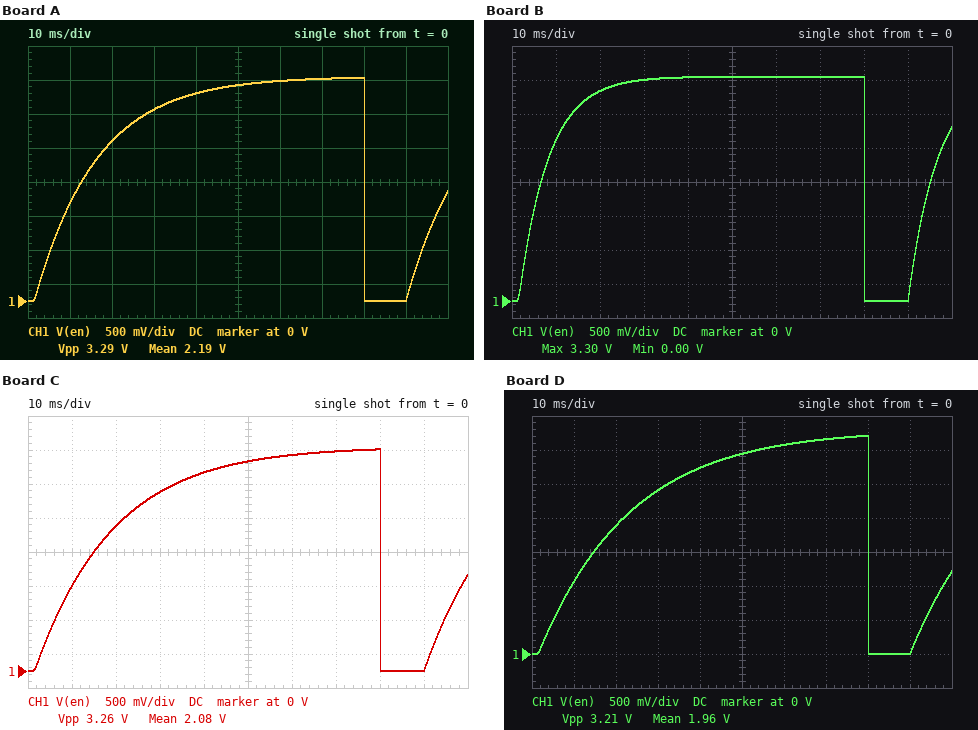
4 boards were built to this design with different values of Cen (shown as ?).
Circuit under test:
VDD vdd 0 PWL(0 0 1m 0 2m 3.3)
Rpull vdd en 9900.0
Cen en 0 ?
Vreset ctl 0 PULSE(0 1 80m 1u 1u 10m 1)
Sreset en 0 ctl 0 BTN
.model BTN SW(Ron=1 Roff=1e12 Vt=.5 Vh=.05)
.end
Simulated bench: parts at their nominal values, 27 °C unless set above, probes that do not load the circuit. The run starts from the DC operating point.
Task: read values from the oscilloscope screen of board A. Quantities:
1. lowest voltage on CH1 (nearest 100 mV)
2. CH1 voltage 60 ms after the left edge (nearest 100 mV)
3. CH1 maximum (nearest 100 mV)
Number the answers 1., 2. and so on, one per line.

1. 0 V
2. 3.2 V
3. 3.3 V
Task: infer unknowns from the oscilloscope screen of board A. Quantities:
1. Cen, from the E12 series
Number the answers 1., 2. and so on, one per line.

1. 1.5 µF
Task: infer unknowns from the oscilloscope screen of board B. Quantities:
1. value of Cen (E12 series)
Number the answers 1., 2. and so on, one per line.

1. 680 nF
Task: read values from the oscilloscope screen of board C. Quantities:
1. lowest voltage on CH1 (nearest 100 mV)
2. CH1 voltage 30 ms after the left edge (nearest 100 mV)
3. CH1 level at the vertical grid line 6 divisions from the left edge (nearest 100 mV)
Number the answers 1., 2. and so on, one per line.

1. 0 V
2. 2.6 V
3. 3.2 V
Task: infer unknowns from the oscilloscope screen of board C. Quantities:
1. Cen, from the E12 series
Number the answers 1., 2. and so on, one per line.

1. 1.8 µF
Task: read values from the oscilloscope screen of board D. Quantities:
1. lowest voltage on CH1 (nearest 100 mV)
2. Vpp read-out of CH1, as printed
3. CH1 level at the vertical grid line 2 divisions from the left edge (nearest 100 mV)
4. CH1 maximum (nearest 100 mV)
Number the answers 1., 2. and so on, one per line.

1. 0 V
2. 3.21 V
3. 1.9 V
4. 3.2 V
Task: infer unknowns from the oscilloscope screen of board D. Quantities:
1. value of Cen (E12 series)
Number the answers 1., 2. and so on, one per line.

1. 2.2 µF
